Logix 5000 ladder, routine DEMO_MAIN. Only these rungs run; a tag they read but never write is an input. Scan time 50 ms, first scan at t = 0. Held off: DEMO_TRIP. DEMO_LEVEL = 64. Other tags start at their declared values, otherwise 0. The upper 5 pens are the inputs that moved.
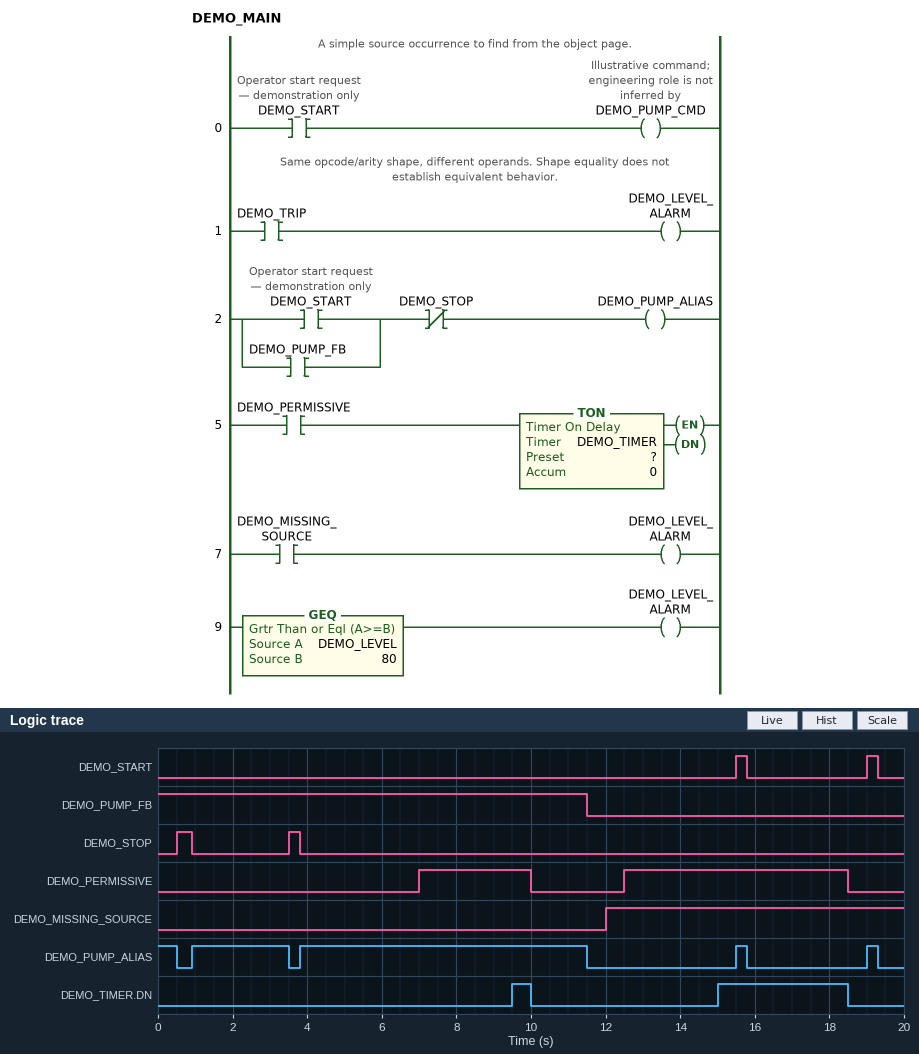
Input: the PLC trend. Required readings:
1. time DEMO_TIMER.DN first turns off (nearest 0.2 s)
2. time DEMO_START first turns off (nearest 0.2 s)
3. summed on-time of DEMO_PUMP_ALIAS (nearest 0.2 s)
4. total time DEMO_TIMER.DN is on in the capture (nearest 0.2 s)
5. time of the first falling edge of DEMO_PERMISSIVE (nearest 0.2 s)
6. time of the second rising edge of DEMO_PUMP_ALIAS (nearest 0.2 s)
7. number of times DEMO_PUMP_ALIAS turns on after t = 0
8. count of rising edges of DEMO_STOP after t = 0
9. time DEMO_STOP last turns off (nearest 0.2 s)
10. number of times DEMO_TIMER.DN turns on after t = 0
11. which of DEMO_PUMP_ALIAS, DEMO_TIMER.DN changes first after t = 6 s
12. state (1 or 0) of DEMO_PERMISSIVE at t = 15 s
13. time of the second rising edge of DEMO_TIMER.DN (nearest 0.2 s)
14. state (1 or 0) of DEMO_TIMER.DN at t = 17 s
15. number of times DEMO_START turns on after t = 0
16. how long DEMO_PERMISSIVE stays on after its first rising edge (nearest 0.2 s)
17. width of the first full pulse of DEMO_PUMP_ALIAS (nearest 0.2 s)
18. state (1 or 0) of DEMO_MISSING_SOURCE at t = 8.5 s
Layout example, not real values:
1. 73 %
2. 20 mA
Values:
1. 10.0 s
2. 15.8 s
3. 11.4 s
4. 4.0 s
5. 10.0 s
6. 3.8 s
7. 4
8. 2
9. 3.8 s
10. 2
11. DEMO_TIMER.DN
12. 1
13. 15.0 s
14. 1
15. 2
16. 3.0 s
17. 2.6 s
18. 0
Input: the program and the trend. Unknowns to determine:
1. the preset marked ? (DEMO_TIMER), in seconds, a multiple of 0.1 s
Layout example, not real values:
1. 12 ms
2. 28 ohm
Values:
1. 2.5 s
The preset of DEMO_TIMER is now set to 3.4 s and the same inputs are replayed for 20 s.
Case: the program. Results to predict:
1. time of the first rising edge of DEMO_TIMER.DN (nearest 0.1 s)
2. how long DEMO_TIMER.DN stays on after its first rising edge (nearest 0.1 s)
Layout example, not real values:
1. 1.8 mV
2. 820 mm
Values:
1. 15.9 s
2. 2.6 s
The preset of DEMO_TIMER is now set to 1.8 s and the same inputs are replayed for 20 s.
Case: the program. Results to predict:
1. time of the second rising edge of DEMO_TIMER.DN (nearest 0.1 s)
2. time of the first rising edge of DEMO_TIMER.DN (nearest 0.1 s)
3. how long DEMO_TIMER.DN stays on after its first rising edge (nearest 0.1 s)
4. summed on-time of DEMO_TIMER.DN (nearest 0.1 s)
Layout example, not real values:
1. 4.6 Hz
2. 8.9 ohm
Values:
1. 14.3 s
2. 8.8 s
3. 1.2 s
4. 5.4 s
